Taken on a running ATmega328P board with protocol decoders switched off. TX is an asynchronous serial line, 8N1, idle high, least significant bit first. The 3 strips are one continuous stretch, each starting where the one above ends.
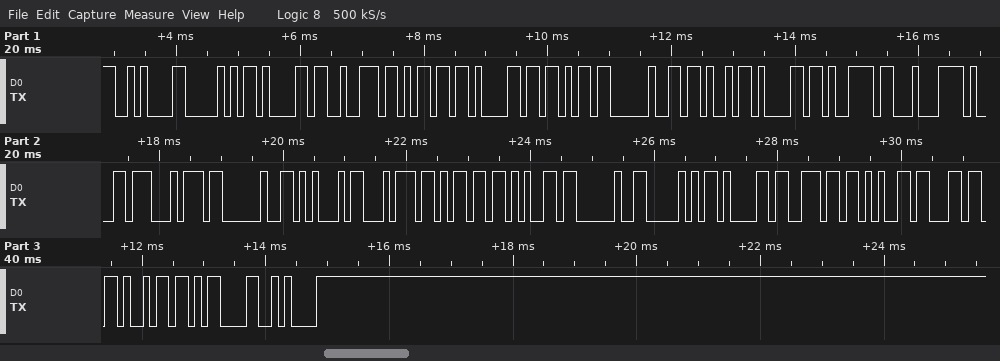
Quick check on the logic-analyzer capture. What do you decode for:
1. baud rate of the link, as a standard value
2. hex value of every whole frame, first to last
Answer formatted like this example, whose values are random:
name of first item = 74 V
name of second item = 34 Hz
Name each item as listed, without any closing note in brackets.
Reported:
baud rate of the link, as a standard value = 9600 baud
hex value of every whole frame, first to last = 0A 50 61 72 6D 61 6B 20 4B 61 79 C4 B1 74 20 45 74 6D 65 20 50 61 6E 65 6C 69 0D 0A
